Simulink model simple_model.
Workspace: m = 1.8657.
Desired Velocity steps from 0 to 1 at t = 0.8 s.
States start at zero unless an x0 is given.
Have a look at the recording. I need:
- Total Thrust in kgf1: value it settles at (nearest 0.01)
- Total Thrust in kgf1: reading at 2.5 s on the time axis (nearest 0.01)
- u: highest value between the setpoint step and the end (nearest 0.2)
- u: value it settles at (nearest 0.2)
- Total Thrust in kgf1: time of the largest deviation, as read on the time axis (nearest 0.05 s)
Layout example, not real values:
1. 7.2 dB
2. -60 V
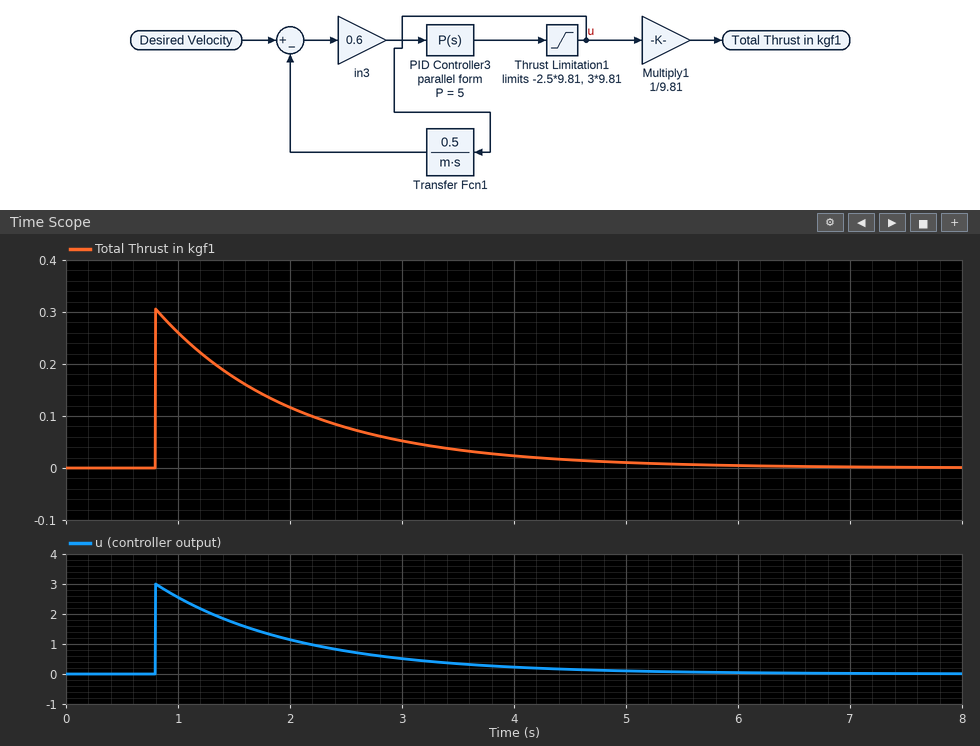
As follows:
1. 0.00
2. 0.08
3. 3.0
4. 0.0
5. 0.80 s
